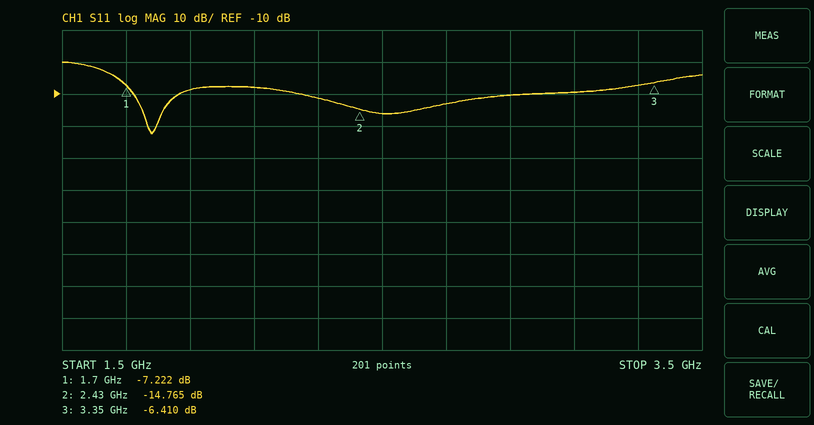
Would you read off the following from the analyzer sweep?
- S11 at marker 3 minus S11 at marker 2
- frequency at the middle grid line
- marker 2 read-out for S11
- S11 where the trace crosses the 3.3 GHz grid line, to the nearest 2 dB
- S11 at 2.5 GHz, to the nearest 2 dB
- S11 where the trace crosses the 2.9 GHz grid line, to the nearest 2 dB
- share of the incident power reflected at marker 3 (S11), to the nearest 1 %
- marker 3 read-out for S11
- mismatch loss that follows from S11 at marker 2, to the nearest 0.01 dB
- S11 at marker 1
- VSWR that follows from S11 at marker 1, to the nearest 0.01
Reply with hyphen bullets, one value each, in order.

- 8.355 dB
- 2.5 GHz
- -14.765 dB
- -8 dB
- -16 dB
- -10 dB
- 23 %
- -6.410 dB
- 0.15 dB
- -7.222 dB
- 2.54
